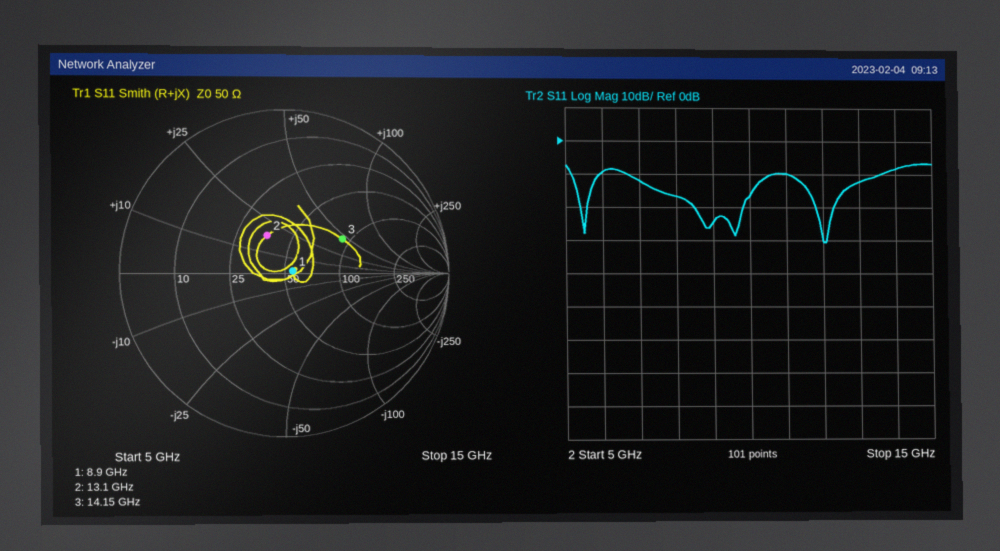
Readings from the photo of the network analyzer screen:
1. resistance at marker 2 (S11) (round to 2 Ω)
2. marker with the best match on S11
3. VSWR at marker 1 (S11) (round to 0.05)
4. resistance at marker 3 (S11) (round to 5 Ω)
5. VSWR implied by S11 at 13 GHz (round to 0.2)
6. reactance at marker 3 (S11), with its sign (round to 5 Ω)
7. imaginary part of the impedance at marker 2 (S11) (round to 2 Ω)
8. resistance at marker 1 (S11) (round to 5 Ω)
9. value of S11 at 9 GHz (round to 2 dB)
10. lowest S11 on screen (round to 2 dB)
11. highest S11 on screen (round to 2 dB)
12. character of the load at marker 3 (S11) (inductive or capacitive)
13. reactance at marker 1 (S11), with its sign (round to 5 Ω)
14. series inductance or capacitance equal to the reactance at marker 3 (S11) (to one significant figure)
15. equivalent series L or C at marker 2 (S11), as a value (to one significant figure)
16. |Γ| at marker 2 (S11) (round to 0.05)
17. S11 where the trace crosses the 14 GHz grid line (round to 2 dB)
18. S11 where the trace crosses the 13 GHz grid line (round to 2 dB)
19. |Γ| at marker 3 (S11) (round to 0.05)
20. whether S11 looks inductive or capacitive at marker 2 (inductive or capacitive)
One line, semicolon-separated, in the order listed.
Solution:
36 Ω; marker 1; 1.10; 90 Ω; 1.6; +45 Ω; +18 Ω; 55 Ω; -24 dB; -30 dB; -6 dB; inductive; 0 Ω; 500 pH; 200 pH; 0.25; -8 dB; -12 dB; 0.40; inductive
